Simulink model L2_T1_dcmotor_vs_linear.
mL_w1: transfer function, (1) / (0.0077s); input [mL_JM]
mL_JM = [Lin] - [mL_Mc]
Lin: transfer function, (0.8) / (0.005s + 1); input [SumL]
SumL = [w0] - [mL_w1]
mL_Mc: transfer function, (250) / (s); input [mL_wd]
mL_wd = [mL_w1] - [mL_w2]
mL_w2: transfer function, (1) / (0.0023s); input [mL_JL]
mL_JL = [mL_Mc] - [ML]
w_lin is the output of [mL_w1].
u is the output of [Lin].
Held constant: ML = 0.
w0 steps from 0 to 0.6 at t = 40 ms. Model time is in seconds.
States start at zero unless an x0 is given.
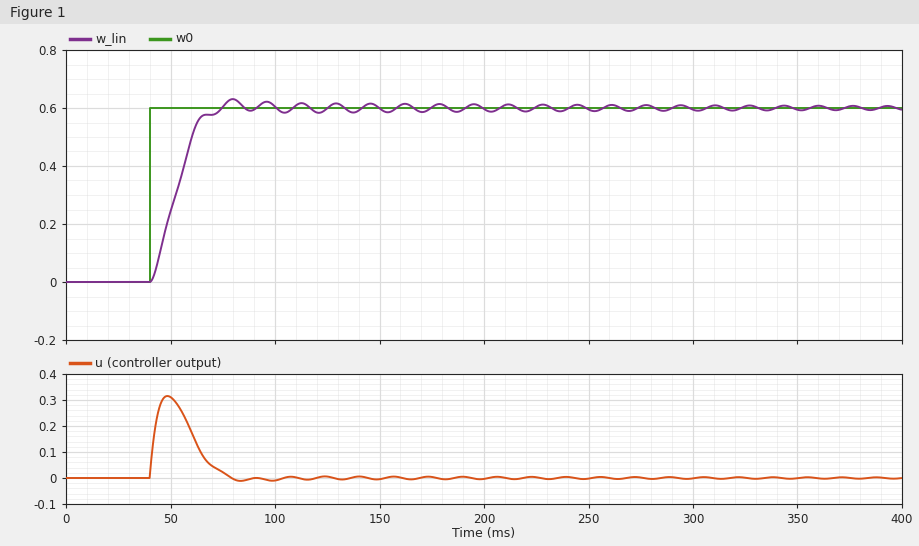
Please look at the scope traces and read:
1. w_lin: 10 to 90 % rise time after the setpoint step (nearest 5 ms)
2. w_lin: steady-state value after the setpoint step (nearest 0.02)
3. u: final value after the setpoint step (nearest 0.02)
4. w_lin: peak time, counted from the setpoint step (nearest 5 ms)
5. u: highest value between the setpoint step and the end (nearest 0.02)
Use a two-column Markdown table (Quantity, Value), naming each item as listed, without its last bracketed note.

| Quantity | Value |
|---|---|
| w_lin: 10 to 90 % rise time after the setpoint step | 20 ms |
| w_lin: steady-state value after the setpoint step | 0.60 |
| u: final value after the setpoint step | 0.00 |
| w_lin: peak time, counted from the setpoint step | 40 ms |
| u: highest value between the setpoint step and the end | 0.32 |
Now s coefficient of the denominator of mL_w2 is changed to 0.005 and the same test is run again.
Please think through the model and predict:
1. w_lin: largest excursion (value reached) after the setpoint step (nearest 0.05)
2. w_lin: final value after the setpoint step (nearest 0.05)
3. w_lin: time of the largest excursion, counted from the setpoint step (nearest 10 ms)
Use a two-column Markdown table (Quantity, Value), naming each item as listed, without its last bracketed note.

| Quantity | Value |
|---|---|
| w_lin: largest excursion (value reached) after the setpoint step | 0.65 |
| w_lin: final value after the setpoint step | 0.60 |
| w_lin: time of the largest excursion, counted from the setpoint step | 50 ms |
